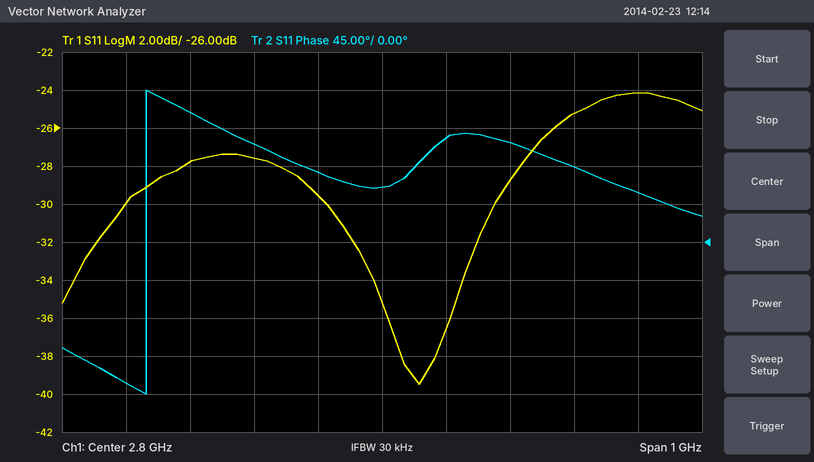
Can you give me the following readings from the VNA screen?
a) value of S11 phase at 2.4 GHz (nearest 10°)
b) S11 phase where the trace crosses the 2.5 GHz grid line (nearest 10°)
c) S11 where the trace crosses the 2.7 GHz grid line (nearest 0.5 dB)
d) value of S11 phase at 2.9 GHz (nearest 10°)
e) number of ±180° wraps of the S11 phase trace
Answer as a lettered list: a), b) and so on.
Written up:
a) -170°
b) 150°
c) -29.5 dB
d) 120°
e) 1
